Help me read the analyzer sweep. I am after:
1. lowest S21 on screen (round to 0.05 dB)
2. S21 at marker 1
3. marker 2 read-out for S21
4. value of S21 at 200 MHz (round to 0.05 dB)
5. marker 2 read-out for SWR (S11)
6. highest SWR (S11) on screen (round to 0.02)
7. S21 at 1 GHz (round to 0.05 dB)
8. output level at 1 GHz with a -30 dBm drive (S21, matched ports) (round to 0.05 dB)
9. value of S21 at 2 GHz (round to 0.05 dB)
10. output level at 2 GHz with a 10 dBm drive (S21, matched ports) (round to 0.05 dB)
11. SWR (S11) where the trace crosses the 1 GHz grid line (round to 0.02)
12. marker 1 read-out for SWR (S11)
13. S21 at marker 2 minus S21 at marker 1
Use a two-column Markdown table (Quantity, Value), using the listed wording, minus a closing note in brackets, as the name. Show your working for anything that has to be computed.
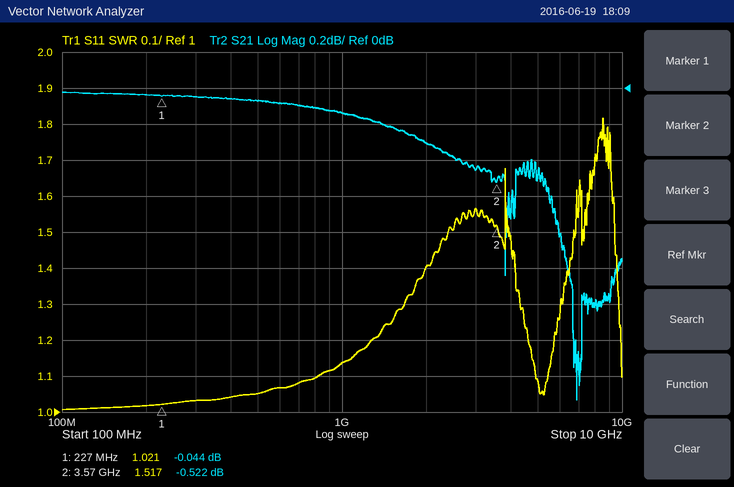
| Quantity | Value |
|---|---|
| lowest S21 on screen | -1.75 dB |
| S21 at marker 1 | -0.044 dB |
| marker 2 read-out for S21 | -0.522 dB |
| value of S21 at 200 MHz | -0.05 dB |
| marker 2 read-out for SWR | 1.517 |
| highest SWR (S11) on screen | 1.82 |
| S21 at 1 GHz | -0.15 dB |
| output level at 1 GHz with a -30 dBm drive (S21, matched ports) | -30 dBm + (-0.15 dB) = -30.15 dBm |
| value of S21 at 2 GHz | -0.30 dB |
| output level at 2 GHz with a 10 dBm drive (S21, matched ports) | 10 dBm + (-0.30 dB) = 9.70 dBm |
| SWR (S11) where the trace crosses the 1 GHz grid line | 1.14 |
| marker 1 read-out for SWR | 1.021 |
| S21 at marker 2 minus S21 at marker 1 | -0.522 − (-0.044) = -0.478 dB |
